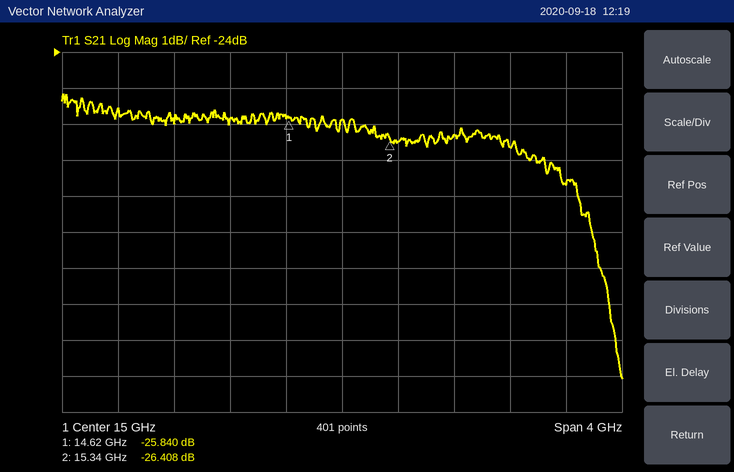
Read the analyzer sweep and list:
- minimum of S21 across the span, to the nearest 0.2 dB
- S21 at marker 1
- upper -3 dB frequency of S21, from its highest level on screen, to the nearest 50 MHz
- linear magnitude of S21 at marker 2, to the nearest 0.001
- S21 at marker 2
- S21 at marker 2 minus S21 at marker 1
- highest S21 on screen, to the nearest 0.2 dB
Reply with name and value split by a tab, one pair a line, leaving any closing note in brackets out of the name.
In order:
minimum of S21 across the span, to the nearest 0.2 dB	-33.0 dB
S21 at marker 1	-25.840 dB
upper -3 dB frequency of S21, from its highest level on screen, to the nearest 50 MHz	16.70 GHz
linear magnitude of S21 at marker 2, to the nearest 0.001	0.048
S21 at marker 2	-26.408 dB
S21 at marker 2 minus S21 at marker 1	-0.568 dB
highest S21 on screen, to the nearest 0.2 dB	-25.2 dB
